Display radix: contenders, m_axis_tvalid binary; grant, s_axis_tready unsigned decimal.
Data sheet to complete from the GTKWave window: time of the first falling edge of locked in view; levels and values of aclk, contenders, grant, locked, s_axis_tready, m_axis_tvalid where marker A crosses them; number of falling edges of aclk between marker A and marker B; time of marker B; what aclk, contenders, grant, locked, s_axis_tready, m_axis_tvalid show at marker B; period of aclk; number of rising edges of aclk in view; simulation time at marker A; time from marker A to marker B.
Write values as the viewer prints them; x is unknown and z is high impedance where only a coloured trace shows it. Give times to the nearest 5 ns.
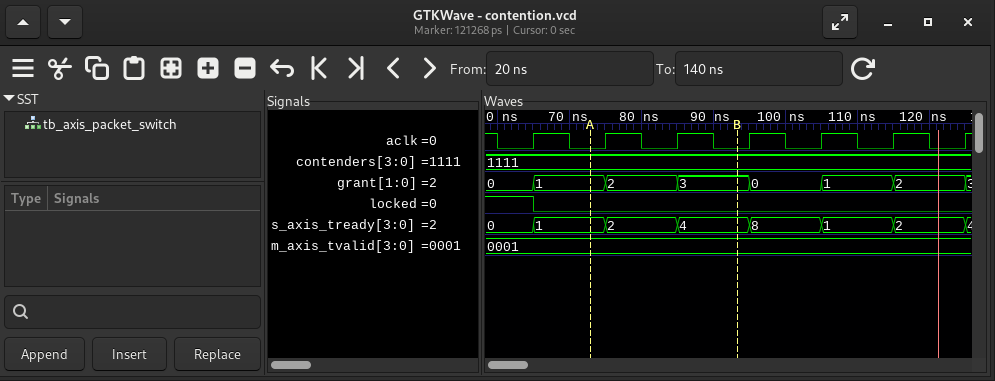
65 ns
aclk=0, contenders=1111, grant=1, locked=0, s_axis_tready=1, m_axis_tvalid=0001
2
95 ns
aclk=0, contenders=1111, grant=3, locked=0, s_axis_tready=4, m_axis_tvalid=0001
10 ns
7
75 ns
20 ns
